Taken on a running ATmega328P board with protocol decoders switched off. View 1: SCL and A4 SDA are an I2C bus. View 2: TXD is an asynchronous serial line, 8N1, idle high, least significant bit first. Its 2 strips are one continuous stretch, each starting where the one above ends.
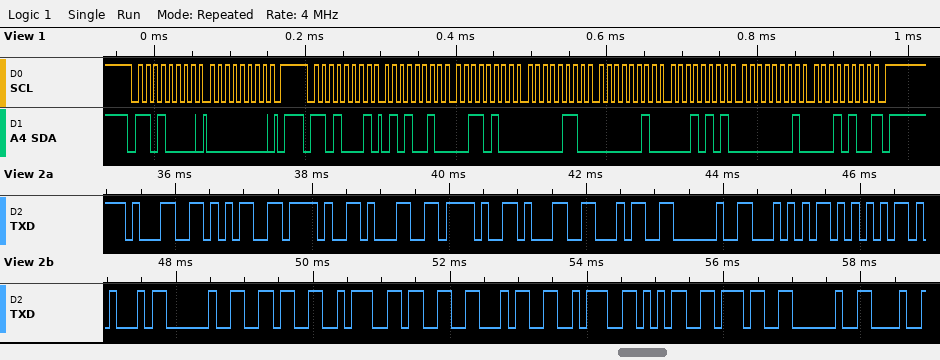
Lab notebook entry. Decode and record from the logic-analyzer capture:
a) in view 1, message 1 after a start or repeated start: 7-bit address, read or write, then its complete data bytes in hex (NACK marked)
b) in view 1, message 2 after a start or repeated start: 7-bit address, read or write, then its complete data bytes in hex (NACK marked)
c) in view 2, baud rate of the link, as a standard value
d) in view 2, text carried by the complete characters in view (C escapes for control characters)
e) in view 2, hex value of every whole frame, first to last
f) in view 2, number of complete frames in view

0x68 write: 00
0x68 read: 52 34 06 02 15 01 14 NACK
9600 baud
"15/1/14 TUE 6:34:57 "
31 35 2F 31 2F 31 34 20 54 55 45 20 36 3A 33 34 3A 35 37 20
20
